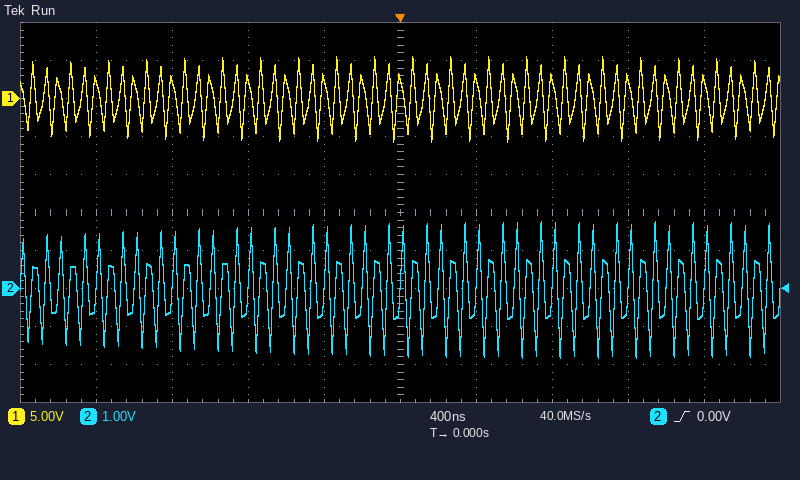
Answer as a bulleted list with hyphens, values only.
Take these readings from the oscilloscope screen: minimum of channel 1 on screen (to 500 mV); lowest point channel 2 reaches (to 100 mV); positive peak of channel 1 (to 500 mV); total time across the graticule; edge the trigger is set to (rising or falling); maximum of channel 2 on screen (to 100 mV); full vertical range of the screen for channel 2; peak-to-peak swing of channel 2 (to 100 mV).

- -5.5 V
- -1.8 V
- 5.5 V
- 4 µs
- rising
- 1.8 V
- 10 V
- 3.6 V
